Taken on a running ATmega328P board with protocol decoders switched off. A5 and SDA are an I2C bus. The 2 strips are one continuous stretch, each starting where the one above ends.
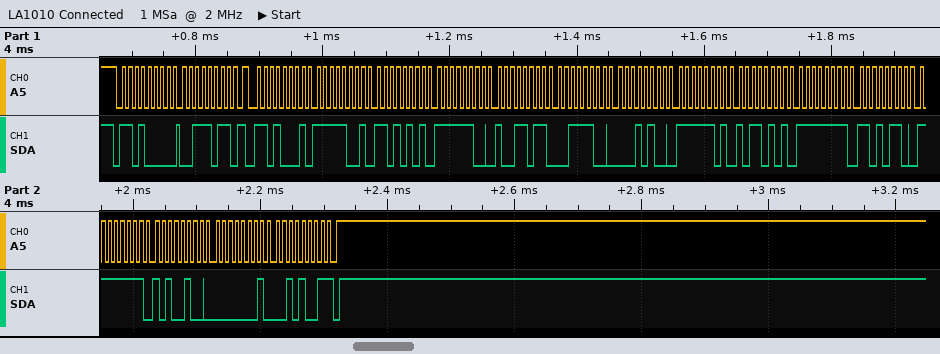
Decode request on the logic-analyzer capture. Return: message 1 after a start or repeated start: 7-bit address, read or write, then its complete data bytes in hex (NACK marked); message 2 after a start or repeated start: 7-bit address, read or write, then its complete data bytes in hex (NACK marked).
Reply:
0x68 write: 3B
0x68 read: F9 D5 FC 9B 3C 14 FD B5 FF D6 FF A4 01 29 NACK
